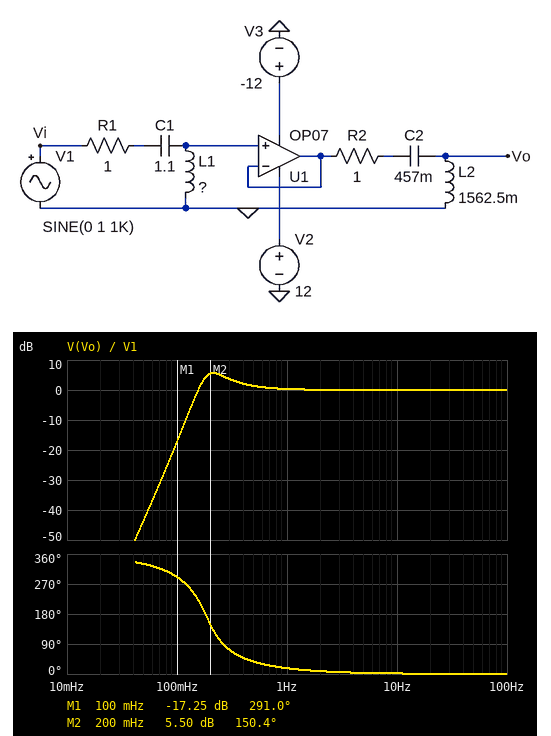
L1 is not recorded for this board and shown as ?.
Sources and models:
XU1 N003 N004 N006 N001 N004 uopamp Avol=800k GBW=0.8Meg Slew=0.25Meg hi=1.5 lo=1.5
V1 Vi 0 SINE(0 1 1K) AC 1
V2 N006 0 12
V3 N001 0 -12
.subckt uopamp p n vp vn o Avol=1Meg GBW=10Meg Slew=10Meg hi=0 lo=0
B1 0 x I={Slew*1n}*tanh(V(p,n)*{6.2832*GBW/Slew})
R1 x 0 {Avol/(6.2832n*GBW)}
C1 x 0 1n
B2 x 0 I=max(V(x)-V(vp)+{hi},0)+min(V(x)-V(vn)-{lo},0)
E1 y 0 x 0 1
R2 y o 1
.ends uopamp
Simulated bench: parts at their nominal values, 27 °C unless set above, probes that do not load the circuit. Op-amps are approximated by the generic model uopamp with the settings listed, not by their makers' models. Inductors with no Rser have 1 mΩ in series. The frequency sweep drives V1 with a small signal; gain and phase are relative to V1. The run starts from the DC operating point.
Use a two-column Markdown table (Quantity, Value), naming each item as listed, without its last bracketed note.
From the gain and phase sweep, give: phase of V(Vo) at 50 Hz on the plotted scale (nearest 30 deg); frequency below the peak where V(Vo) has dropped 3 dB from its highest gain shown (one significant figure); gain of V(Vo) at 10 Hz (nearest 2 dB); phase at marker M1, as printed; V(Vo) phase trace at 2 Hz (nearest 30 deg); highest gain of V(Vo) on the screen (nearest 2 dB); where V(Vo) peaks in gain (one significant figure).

| Quantity | Value |
|---|---|
| phase of V(Vo) at 50 Hz on the plotted scale | 0 deg |
| frequency below the peak where V(Vo) has dropped 3 dB from its highest gain shown | 200 mHz |
| gain of V(Vo) at 10 Hz | 0 dB |
| phase at marker M1, as printed | 291.0 deg |
| V(Vo) phase trace at 2 Hz | 0 deg |
| highest gain of V(Vo) on the screen | 6 dB |
| where V(Vo) peaks in gain | 200 mHz |
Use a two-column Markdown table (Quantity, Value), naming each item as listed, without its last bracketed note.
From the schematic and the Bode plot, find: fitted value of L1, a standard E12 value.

| Quantity | Value |
|---|---|
| fitted value of L1, a standard E12 value | 820 mH |
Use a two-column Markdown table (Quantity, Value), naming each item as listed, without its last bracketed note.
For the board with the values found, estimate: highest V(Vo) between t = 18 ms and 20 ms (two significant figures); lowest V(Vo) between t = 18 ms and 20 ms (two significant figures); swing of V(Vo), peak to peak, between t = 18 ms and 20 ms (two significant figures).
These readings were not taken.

| Quantity | Value |
|---|---|
| highest V(Vo) between t = 18 ms and 20 ms | 1.0 V |
| lowest V(Vo) between t = 18 ms and 20 ms | -1.0 V |
| swing of V(Vo), peak to peak, between t = 18 ms and 20 ms | 2.0 V |
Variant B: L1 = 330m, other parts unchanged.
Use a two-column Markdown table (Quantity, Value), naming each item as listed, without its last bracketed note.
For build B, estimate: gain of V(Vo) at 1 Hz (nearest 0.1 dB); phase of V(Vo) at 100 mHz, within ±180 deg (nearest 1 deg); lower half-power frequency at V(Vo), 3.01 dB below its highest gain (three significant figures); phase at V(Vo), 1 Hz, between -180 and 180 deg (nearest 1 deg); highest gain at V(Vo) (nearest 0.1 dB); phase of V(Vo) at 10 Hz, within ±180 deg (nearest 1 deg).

| Quantity | Value |
|---|---|
| gain of V(Vo) at 1 Hz | -0.1 dB |
| phase of V(Vo) at 100 mHz, within ±180 deg | -61 deg |
| lower half-power frequency at V(Vo), 3.01 dB below its highest gain | 192 mHz |
| phase at V(Vo), 1 Hz, between -180 and 180 deg | 33 deg |
| highest gain at V(Vo) | 0 dB |
| phase of V(Vo) at 10 Hz, within ±180 deg | 3 deg |
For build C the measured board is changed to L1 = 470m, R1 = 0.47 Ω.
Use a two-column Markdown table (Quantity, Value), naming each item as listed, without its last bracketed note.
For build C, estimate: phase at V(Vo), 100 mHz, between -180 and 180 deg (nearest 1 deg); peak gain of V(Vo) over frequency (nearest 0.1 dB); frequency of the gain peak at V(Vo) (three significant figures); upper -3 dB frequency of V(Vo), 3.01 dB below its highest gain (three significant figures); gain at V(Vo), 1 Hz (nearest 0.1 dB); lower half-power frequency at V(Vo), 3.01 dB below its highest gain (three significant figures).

| Quantity | Value |
|---|---|
| phase at V(Vo), 100 mHz, between -180 and 180 deg | -44 deg |
| peak gain of V(Vo) over frequency | 8.3 dB |
| frequency of the gain peak at V(Vo) | 228 mHz |
| upper -3 dB frequency of V(Vo), 3.01 dB below its highest gain | 331 mHz |
| gain at V(Vo), 1 Hz | 0.6 dB |
| lower half-power frequency at V(Vo), 3.01 dB below its highest gain | 184 mHz |
